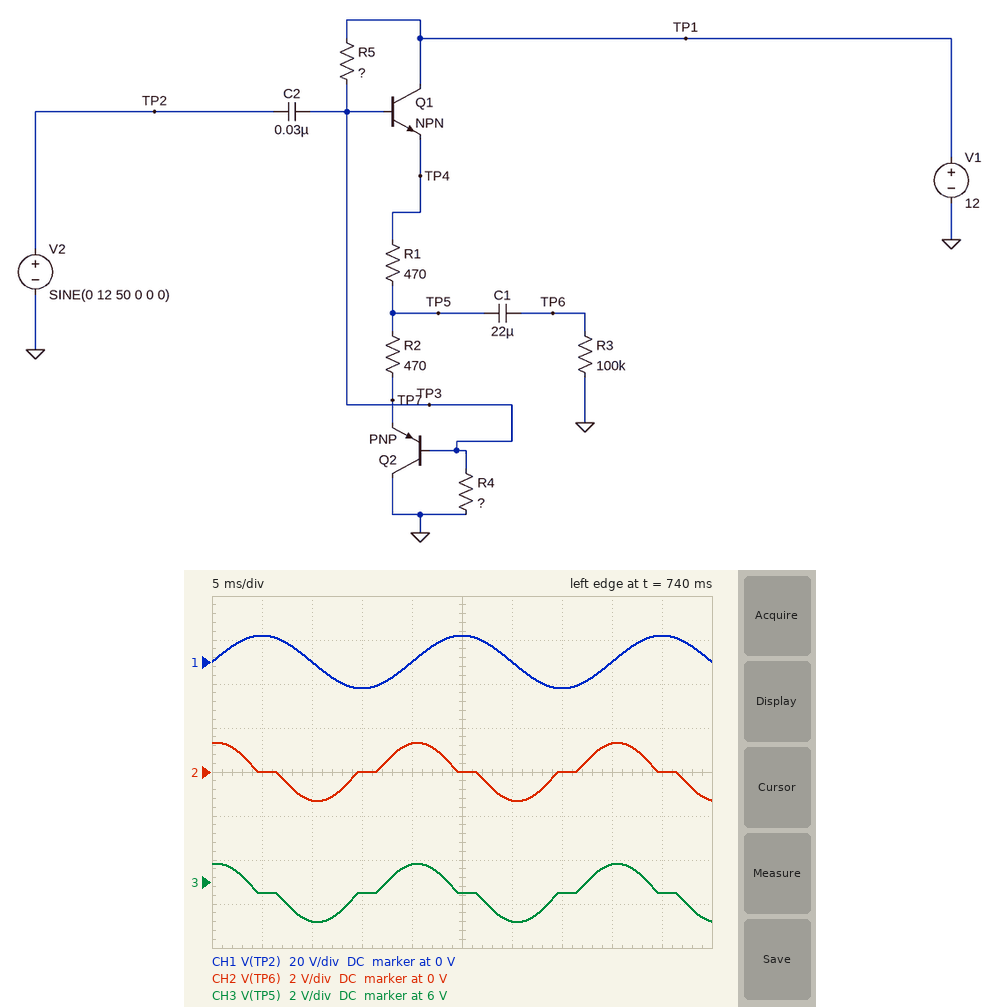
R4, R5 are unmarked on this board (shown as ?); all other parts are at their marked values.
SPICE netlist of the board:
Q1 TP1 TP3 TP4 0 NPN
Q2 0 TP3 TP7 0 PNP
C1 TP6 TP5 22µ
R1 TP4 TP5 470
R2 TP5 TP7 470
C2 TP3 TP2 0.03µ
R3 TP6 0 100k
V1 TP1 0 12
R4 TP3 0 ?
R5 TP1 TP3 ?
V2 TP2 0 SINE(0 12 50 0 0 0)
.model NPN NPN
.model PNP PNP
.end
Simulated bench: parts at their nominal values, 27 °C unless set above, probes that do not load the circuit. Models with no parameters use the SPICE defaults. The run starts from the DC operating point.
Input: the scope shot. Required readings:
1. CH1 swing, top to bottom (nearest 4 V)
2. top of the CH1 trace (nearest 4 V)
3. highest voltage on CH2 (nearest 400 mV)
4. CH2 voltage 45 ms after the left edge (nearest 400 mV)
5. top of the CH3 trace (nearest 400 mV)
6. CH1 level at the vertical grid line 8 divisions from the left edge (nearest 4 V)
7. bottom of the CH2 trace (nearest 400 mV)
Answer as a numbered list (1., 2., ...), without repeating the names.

1. 24 V
2. 12 V
3. 1.2 V
4. 0 V
5. 6.8 V
6. 0 V
7. -1.2 V
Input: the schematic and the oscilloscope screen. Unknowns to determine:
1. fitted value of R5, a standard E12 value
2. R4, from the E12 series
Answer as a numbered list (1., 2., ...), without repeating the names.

1. 39 kΩ
2. 33 kΩ
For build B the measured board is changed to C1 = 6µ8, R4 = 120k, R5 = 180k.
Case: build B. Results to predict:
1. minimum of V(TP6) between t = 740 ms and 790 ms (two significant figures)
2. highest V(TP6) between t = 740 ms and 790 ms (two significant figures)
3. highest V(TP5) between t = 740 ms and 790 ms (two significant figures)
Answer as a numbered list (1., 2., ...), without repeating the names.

1. -4.9 V
2. 5.8 V
3. 11 V
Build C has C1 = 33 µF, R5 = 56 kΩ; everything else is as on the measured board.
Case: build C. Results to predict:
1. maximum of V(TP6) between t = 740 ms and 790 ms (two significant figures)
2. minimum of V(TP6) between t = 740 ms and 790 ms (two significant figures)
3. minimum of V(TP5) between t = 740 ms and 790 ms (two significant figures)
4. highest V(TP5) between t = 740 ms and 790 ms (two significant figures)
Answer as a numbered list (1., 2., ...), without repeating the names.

1. 1.6 V
2. -1.6 V
3. 2.8 V
4. 6.1 V
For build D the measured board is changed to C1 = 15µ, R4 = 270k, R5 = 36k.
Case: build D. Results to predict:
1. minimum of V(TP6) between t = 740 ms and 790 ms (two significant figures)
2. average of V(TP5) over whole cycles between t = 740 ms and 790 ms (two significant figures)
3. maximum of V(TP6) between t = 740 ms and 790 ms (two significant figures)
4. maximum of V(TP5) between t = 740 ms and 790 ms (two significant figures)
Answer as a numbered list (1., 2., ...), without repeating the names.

1. -2.6 V
2. 10 V
3. 1.5 V
4. 12 V
